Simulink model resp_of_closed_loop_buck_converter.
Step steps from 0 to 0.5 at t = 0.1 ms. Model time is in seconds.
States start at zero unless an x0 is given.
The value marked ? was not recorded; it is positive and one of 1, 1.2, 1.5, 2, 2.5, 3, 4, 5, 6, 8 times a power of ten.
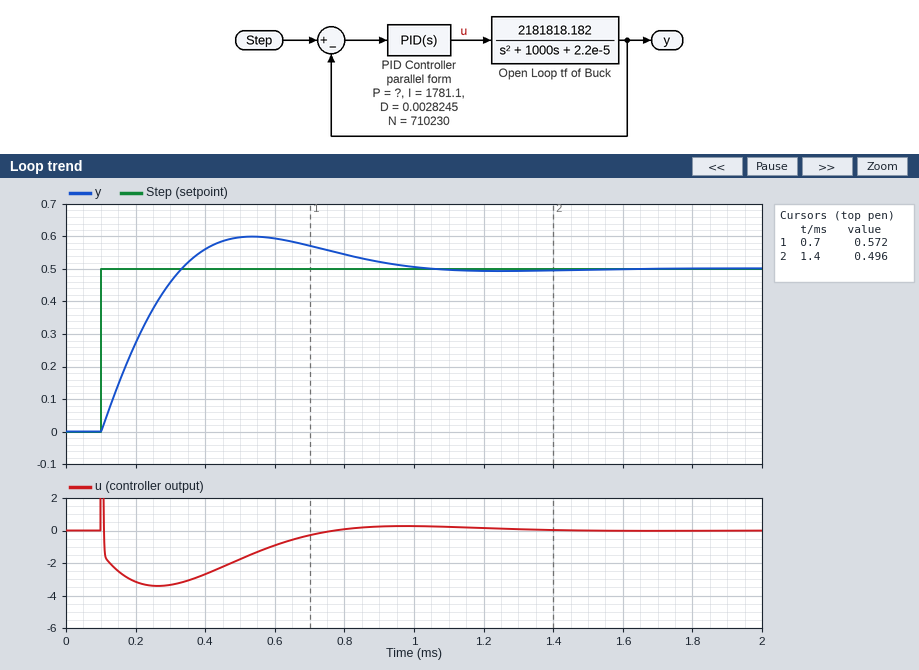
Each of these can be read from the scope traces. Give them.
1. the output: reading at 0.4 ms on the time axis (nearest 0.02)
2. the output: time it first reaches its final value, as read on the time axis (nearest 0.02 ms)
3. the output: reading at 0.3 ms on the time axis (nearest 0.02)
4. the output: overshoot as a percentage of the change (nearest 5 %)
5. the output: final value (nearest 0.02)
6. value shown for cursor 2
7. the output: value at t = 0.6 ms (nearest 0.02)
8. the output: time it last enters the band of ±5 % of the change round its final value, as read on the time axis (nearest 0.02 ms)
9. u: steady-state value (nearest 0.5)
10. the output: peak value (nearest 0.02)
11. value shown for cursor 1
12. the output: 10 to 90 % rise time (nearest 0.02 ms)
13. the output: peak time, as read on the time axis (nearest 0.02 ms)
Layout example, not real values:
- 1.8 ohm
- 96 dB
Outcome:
- 0.56
- 0.34 ms
- 0.46
- 20 %
- 0.50
- 0.496
- 0.60
- 0.88 ms
- 0.0
- 0.60
- 0.572
- 0.18 ms
- 0.54 ms
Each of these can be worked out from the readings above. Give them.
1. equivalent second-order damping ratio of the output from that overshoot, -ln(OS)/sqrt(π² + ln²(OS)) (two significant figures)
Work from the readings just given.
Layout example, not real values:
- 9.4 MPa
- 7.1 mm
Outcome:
- 0.46
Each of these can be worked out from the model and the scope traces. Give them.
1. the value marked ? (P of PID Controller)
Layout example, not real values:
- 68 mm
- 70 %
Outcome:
- 15
